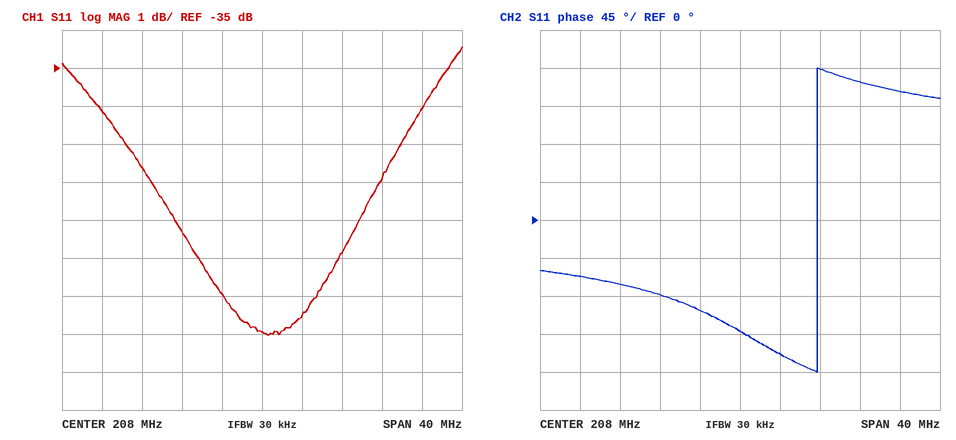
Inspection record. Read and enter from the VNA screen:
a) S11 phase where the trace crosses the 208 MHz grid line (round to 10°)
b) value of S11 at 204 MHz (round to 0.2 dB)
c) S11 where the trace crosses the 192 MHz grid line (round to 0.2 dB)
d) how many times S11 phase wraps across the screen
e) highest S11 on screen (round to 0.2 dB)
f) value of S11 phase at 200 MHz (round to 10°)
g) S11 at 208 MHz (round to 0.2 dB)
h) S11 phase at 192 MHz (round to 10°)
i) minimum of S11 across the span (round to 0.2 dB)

-130°
-41.0 dB
-36.2 dB
1
-34.4 dB
-90°
-42.0 dB
-70°
-42.0 dB
